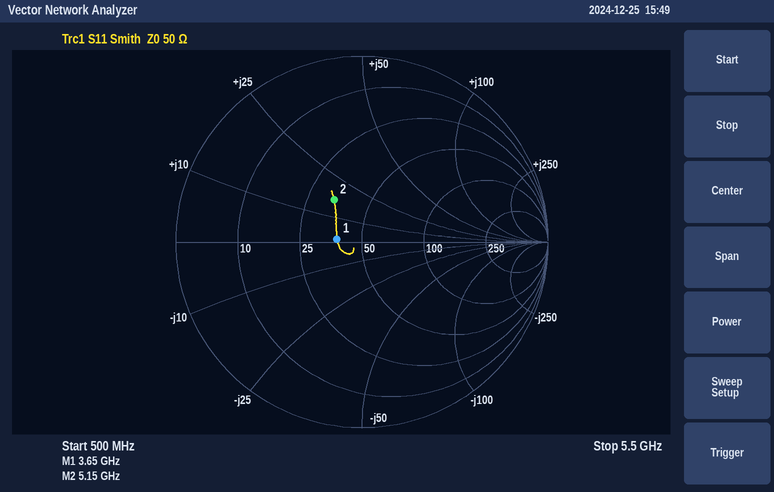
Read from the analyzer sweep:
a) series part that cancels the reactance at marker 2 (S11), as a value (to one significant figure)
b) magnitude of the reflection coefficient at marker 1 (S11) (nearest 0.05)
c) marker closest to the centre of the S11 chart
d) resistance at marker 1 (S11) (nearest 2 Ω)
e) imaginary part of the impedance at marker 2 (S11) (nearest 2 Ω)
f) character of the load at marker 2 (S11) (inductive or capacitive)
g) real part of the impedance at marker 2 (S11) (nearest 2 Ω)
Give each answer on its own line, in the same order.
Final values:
2 pF
0.15
marker 1
38 Ω
+16 Ω
inductive
34 Ω
